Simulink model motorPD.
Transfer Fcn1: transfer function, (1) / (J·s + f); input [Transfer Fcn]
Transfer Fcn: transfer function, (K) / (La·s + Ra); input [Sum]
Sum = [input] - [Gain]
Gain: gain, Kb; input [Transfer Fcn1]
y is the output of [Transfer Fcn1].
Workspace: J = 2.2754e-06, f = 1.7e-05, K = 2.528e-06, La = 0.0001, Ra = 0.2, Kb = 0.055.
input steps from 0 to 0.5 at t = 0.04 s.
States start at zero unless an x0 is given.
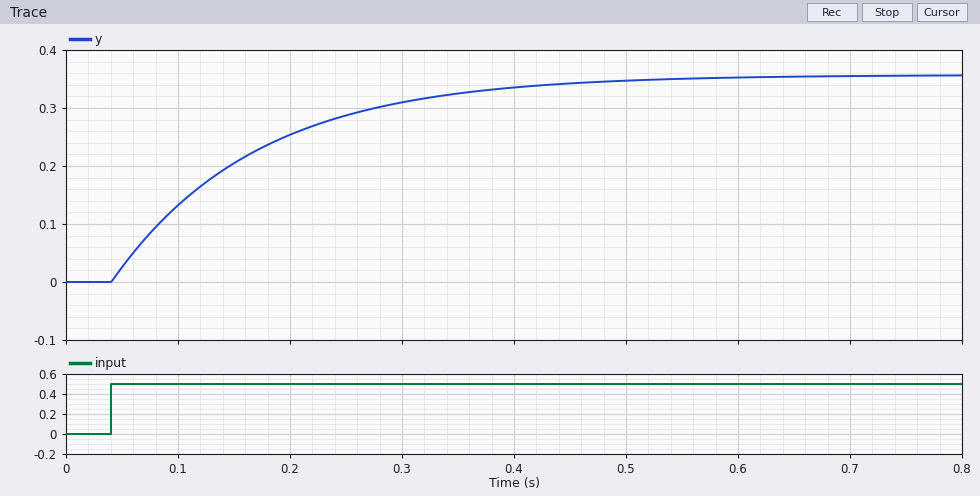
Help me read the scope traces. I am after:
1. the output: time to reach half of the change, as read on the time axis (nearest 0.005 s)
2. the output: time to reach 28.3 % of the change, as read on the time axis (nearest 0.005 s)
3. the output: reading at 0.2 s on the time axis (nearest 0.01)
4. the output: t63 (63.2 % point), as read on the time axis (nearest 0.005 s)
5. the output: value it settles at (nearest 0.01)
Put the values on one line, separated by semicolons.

0.130 s; 0.085 s; 0.25; 0.170 s; 0.36
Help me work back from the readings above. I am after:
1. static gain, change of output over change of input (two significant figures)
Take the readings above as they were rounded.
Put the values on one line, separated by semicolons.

0.72
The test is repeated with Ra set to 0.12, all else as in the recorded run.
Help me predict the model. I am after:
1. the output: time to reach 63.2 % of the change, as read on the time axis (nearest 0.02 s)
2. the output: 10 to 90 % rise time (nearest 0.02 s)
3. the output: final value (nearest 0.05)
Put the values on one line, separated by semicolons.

0.16 s; 0.28 s; 0.60
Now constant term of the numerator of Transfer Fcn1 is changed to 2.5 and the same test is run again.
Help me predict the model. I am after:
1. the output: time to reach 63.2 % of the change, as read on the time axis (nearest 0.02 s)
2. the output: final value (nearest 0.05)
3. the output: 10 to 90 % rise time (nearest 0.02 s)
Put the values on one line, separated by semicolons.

0.16 s; 0.85; 0.26 s
